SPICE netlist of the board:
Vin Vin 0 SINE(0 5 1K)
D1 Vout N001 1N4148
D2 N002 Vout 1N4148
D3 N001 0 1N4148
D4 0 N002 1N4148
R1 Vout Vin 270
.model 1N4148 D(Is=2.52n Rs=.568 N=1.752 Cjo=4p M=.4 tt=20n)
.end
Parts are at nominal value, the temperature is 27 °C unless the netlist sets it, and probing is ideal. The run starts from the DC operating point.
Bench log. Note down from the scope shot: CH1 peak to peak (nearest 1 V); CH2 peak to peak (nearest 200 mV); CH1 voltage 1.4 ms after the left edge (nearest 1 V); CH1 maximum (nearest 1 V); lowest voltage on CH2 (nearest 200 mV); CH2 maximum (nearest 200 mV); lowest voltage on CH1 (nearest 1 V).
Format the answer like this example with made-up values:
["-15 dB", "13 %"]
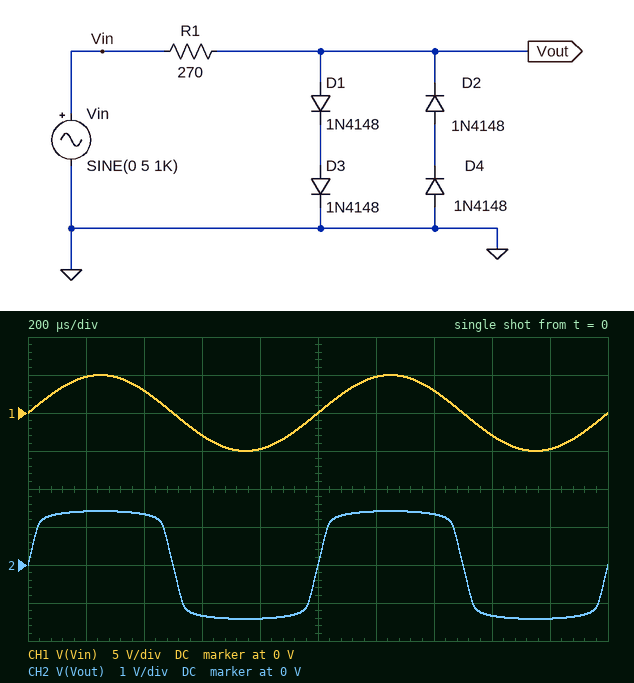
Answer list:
["10 V", "2.8 V", "3 V", "5 V", "-1.4 V", "1.4 V", "-5 V"]
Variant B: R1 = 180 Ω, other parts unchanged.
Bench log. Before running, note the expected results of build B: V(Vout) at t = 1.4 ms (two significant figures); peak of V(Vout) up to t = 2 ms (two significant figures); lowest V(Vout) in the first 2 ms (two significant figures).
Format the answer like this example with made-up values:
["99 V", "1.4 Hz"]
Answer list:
["1.4 V", "1.5 V", "-1.5 V"]
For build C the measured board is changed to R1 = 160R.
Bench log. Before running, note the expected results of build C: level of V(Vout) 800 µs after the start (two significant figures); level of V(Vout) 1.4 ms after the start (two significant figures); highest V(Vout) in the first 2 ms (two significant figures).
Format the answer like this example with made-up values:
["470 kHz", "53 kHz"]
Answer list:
["-1.5 V", "1.4 V", "1.5 V"]
